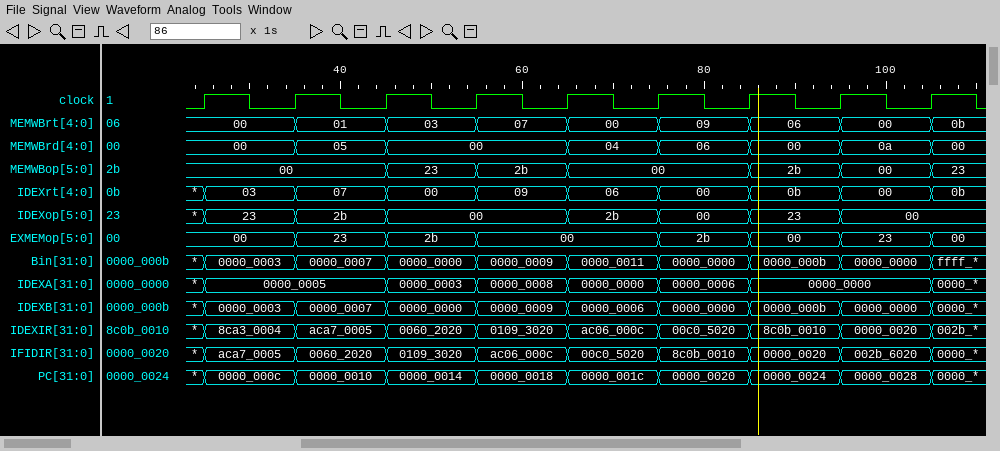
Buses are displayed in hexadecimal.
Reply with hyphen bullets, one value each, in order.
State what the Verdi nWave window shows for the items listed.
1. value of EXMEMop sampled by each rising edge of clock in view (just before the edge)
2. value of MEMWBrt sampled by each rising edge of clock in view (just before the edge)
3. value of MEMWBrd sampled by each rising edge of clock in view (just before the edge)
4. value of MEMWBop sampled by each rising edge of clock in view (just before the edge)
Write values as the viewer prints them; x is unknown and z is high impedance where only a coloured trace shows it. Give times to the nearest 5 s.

- 00, 00, 23, 2b, 00, 00, 2b, 00, 23
- 00, 00, 01, 03, 07, 00, 09, 06, 00
- 00, 00, 05, 00, 00, 04, 06, 00, 0a
- 00, 00, 00, 23, 2b, 00, 00, 2b, 00
